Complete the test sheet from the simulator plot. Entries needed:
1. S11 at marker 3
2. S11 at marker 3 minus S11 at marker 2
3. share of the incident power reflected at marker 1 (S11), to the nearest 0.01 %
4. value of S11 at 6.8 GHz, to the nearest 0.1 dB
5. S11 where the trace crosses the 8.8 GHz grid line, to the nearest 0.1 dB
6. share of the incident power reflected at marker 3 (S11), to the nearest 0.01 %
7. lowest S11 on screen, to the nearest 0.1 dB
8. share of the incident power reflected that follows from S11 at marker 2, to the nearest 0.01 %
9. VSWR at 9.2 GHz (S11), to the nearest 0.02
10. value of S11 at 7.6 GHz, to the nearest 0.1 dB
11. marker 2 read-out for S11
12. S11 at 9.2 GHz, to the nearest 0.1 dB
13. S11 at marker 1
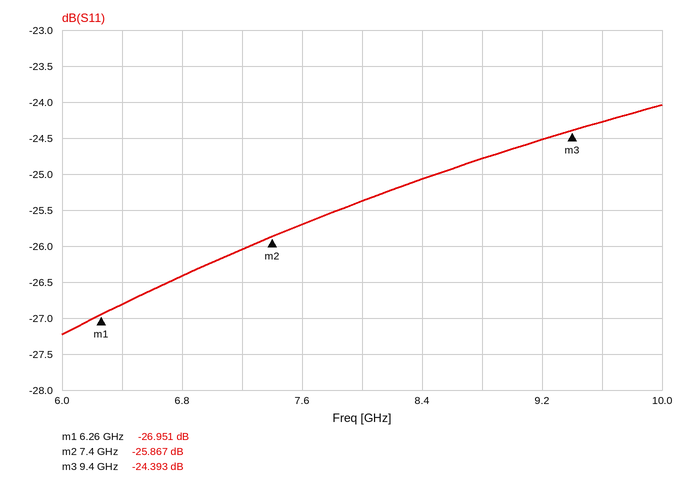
-24.393 dB
1.474 dB
0.20 %
-26.4 dB
-24.8 dB
0.36 %
-27.2 dB
0.26 %
1.12
-25.7 dB
-25.867 dB
-24.5 dB
-26.951 dB
